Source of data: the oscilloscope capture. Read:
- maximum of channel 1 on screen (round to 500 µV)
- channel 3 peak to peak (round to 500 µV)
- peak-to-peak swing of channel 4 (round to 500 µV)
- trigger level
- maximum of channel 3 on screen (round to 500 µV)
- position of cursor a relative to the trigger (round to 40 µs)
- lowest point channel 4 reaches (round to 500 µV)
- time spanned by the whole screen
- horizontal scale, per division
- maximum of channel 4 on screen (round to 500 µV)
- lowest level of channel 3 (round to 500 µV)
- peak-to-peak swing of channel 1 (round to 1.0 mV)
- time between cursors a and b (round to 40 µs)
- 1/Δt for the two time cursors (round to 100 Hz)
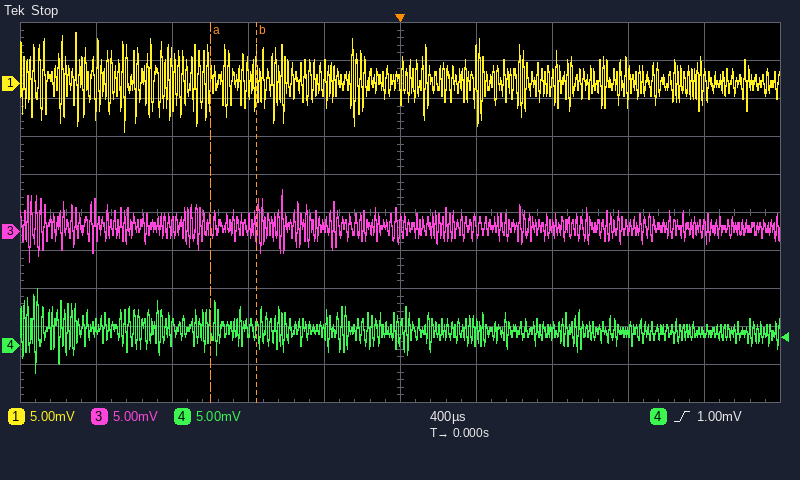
6.5 mV
9.5 mV
11.0 mV
1.00 mV
5.5 mV
-1.00 ms
-3.5 mV
4 ms
400 µs
7.5 mV
-4.0 mV
13.0 mV
240 µs
4.2 kHz
